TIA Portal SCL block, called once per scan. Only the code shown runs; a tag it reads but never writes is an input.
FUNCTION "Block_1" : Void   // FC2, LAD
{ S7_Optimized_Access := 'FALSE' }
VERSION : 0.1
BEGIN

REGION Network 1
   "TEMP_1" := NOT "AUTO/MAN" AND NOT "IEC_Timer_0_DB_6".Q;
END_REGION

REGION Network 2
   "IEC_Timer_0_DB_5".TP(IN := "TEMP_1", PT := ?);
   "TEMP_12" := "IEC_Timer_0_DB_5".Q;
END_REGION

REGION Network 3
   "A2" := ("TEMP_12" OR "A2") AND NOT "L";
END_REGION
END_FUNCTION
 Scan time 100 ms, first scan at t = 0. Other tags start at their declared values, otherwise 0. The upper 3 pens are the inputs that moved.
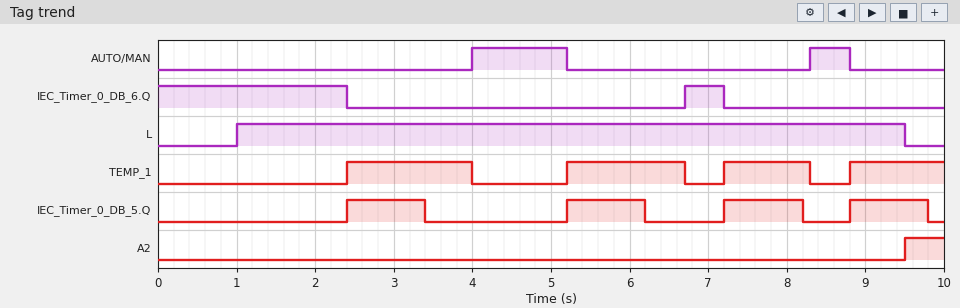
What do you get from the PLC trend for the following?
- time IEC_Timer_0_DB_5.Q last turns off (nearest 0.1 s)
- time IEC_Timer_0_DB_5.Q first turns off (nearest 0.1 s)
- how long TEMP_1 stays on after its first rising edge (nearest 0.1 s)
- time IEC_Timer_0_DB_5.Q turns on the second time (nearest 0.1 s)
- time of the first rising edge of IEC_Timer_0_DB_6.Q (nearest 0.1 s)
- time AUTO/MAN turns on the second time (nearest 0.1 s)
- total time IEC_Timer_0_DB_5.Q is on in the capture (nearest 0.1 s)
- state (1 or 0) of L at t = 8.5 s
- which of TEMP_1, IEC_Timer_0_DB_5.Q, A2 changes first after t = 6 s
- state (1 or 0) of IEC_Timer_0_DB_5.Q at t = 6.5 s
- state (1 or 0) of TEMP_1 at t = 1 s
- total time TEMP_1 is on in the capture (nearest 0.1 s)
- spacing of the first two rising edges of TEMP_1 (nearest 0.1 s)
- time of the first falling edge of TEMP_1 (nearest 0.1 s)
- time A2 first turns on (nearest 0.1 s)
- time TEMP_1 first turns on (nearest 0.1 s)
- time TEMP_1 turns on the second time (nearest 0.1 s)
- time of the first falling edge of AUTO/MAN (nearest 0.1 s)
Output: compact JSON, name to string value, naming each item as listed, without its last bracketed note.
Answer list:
{"time IEC_Timer_0_DB_5.Q last turns off": "9.8 s", "time IEC_Timer_0_DB_5.Q first turns off": "3.4 s", "how long TEMP_1 stays on after its first rising edge": "1.6 s", "time IEC_Timer_0_DB_5.Q turns on the second time": "5.2 s", "time of the first rising edge of IEC_Timer_0_DB_6.Q": "6.7 s", "time AUTO/MAN turns on the second time": "8.3 s", "total time IEC_Timer_0_DB_5.Q is on in the capture": "4.0 s", "state (1 or 0) of L at t = 8.5 s": "1", "which of TEMP_1, IEC_Timer_0_DB_5.Q, A2 changes first after t = 6 s": "IEC_Timer_0_DB_5.Q", "state (1 or 0) of IEC_Timer_0_DB_5.Q at t = 6.5 s": "0", "state (1 or 0) of TEMP_1 at t = 1 s": "0", "total time TEMP_1 is on in the capture": "5.4 s", "spacing of the first two rising edges of TEMP_1": "2.8 s", "time of the first falling edge of TEMP_1": "4.0 s", "time A2 first turns on": "9.5 s", "time TEMP_1 first turns on": "2.4 s", "time TEMP_1 turns on the second time": "5.2 s", "time of the first falling edge of AUTO/MAN": "5.2 s"}
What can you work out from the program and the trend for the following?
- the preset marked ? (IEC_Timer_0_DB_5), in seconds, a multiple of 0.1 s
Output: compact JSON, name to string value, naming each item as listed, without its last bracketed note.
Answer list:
{"the preset marked ? (IEC_Timer_0_DB_5), in seconds, a multiple of 0.1 s": "1.0 s"}
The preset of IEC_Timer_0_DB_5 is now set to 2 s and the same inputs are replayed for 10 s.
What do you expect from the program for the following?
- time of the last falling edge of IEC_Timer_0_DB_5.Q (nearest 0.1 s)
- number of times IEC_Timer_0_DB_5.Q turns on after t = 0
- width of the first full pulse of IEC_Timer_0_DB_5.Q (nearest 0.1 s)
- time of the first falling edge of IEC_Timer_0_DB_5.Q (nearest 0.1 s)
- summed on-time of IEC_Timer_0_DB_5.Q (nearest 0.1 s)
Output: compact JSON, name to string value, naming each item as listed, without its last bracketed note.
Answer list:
{"time of the last falling edge of IEC_Timer_0_DB_5.Q": "7.2 s", "number of times IEC_Timer_0_DB_5.Q turns on after t = 0": "3", "width of the first full pulse of IEC_Timer_0_DB_5.Q": "2.0 s", "time of the first falling edge of IEC_Timer_0_DB_5.Q": "4.4 s", "summed on-time of IEC_Timer_0_DB_5.Q": "5.2 s"}
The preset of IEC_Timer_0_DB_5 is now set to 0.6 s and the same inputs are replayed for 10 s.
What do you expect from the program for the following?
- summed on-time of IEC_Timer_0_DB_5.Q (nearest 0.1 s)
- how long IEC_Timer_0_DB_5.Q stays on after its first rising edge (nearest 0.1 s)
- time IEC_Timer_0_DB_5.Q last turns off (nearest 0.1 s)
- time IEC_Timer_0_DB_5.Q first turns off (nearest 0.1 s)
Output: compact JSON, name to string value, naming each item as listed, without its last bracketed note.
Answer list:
{"summed on-time of IEC_Timer_0_DB_5.Q": "2.4 s", "how long IEC_Timer_0_DB_5.Q stays on after its first rising edge": "0.6 s", "time IEC_Timer_0_DB_5.Q last turns off": "9.4 s", "time IEC_Timer_0_DB_5.Q first turns off": "3.0 s"}
